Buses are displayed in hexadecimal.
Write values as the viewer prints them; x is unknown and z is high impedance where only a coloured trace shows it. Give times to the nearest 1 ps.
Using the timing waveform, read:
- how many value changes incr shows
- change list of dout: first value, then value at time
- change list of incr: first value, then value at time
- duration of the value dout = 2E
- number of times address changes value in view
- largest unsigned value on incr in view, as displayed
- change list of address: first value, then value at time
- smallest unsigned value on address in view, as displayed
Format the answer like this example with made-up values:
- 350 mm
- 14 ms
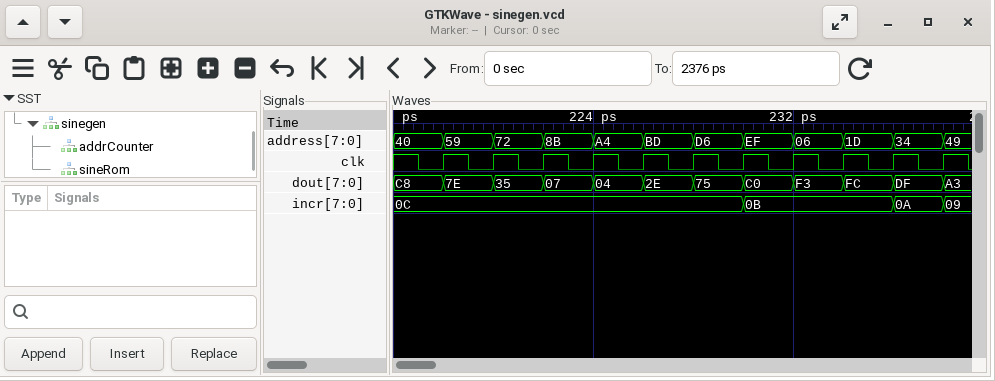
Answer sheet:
- 3
- C8, 7E at 218 ps, 35 at 220 ps, 07 at 222 ps, 04 at 224 ps, 2E at 226 ps, 75 at 228 ps, C0 at 230 ps, F3 at 232 ps, FC at 234 ps, DF at 236 ps, A3 at 238 ps
- 0C, 0B at 230 ps, 0A at 236 ps, 09 at 238 ps
- 2 ps
- 11
- 0C
- 40, 59 at 218 ps, 72 at 220 ps, 8B at 222 ps, A4 at 224 ps, BD at 226 ps, D6 at 228 ps, EF at 230 ps, 06 at 232 ps, 1D at 234 ps, 34 at 236 ps, 49 at 238 ps
- 06
